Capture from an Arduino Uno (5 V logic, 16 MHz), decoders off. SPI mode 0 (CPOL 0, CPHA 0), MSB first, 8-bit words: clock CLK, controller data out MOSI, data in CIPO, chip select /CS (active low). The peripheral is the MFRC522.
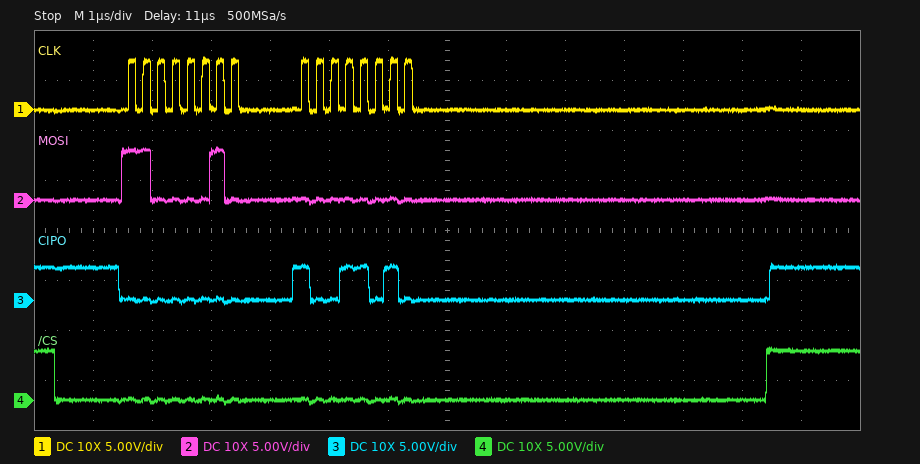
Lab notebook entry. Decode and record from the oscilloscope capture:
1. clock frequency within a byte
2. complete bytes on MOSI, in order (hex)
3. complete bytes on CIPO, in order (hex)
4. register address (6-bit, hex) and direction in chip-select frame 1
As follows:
4 MHz
C2 00
00 9A
0x21 read
